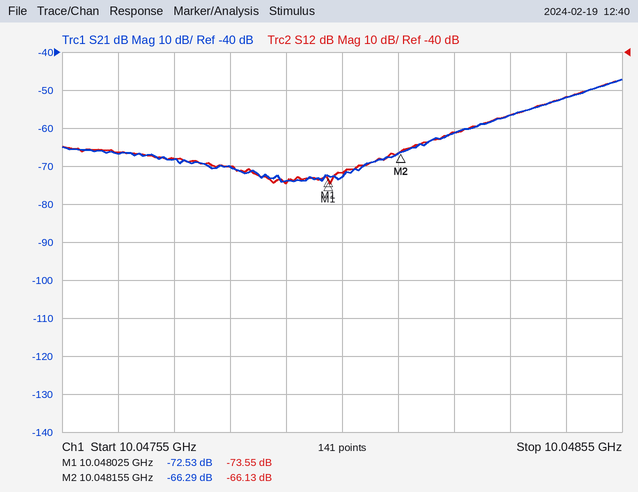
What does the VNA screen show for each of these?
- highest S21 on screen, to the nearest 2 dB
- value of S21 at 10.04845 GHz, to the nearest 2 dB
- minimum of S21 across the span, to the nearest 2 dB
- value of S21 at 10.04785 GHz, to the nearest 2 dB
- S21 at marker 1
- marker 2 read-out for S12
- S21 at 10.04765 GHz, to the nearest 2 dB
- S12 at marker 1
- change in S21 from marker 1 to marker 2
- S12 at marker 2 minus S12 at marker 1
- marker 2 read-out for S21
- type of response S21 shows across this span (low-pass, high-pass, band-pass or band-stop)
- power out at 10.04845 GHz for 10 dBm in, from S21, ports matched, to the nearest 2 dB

-48 dB
-52 dB
-74 dB
-70 dB
-72.53 dB
-66.13 dB
-66 dB
-73.55 dB
6.24 dB
7.42 dB
-66.29 dB
high-pass
-42 dBm
